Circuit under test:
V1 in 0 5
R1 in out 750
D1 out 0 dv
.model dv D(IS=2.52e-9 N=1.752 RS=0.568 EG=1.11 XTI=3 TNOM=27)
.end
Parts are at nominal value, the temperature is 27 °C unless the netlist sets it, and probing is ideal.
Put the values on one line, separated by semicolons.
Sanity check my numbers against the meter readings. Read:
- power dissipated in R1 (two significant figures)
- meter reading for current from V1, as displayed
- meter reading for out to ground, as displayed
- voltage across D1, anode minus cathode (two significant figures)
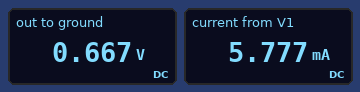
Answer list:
25 mW; 5.777 mA; 0.667 V; 670 mV
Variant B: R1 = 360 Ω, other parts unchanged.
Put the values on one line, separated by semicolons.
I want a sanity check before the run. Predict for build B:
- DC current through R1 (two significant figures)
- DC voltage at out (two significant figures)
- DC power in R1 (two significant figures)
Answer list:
12 mA; 700 mV; 51 mW
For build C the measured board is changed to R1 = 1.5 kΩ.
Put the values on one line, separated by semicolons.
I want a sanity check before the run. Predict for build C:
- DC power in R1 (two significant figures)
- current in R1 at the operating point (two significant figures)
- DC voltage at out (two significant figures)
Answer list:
13 mW; 2.9 mA; 630 mV
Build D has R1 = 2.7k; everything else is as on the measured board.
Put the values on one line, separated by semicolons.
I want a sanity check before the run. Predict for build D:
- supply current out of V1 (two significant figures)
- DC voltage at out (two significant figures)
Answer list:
1.6 mA; 610 mV
